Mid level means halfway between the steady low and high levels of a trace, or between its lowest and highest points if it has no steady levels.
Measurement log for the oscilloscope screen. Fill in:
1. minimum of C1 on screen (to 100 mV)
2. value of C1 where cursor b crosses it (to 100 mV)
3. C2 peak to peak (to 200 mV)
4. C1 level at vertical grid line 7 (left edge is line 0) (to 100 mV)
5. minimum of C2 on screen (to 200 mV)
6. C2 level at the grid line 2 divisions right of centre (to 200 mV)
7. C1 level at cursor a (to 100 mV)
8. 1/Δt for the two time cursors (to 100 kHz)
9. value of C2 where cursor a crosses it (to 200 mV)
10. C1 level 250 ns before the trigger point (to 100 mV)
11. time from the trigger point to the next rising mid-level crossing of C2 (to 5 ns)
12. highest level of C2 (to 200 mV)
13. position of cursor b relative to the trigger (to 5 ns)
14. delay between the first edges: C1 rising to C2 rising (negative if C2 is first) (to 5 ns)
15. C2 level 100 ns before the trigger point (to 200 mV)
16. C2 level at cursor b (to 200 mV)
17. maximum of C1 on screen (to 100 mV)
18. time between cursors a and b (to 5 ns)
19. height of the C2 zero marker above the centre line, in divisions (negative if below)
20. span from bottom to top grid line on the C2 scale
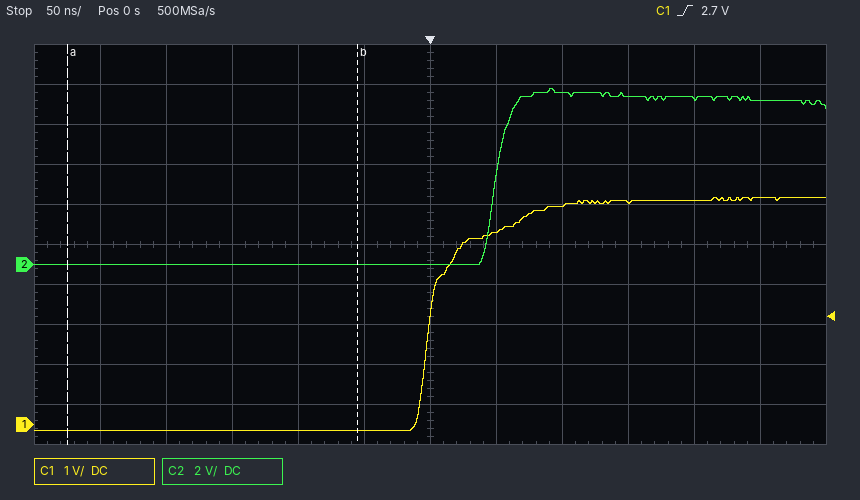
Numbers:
-200 mV
-200 mV
8.8 V
4.8 V
0.0 V
8.6 V
-200 mV
4.5 MHz
0.0 V
-200 mV
50 ns
8.8 V
-55 ns
+50 ns
0.0 V
0.0 V
5.7 V
220 ns
-0.5 div
20 V
